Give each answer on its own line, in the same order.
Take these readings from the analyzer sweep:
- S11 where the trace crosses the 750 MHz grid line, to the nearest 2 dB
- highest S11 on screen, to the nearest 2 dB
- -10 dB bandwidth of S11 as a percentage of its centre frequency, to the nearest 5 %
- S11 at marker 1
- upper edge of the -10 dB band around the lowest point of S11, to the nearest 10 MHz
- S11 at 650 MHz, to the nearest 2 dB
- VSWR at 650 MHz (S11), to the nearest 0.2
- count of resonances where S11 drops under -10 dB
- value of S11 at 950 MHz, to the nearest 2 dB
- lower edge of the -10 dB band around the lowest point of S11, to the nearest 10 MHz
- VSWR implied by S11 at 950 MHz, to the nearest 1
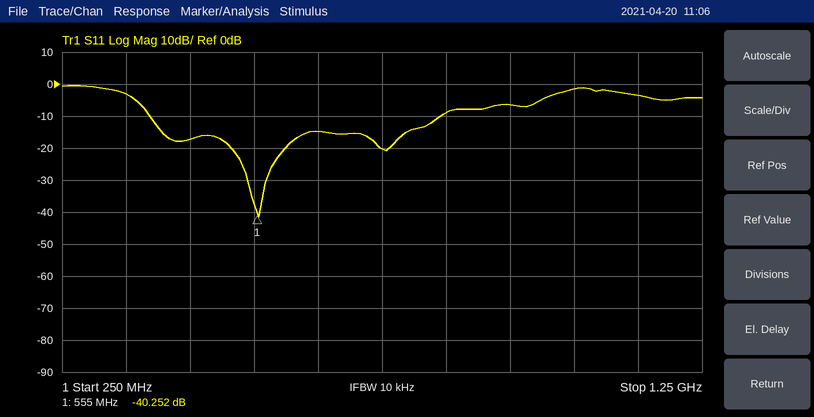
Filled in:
-20 dB
0 dB
75 %
-40.252 dB
840 MHz
-14 dB
1.4
2
-6 dB
390 MHz
3
